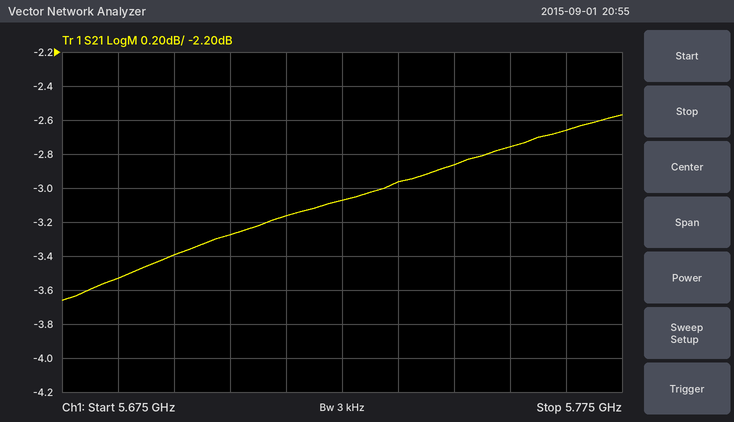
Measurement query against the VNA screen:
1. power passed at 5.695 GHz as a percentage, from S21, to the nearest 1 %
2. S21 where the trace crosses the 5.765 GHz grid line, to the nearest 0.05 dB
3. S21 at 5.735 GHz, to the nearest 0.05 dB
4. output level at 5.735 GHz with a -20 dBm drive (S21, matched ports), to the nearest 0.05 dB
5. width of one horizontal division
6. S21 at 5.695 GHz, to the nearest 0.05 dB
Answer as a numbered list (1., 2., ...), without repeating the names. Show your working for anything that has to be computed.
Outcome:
1. 10^(-3.4/10) ≈ 46 %
2. -2.65 dB
3. -2.95 dB
4. -20 dBm + (-2.95 dB) = -22.95 dBm
5. 10 MHz
6. -3.40 dB
